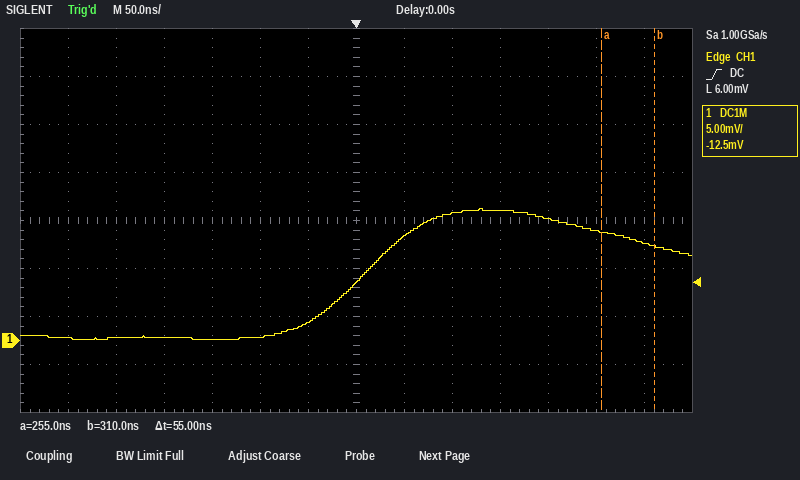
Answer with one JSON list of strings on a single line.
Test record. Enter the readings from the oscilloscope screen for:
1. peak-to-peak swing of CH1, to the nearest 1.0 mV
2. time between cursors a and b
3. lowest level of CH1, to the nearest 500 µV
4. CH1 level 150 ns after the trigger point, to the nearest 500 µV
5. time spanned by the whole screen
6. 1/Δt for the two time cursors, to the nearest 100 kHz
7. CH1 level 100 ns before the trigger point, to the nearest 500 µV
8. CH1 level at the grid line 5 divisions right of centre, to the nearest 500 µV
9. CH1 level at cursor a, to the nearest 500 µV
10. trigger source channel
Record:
["14.0 mV", "55 ns", "0.0 mV", "13.5 mV", "700 ns", "18.2 MHz", "500 µV", "11.5 mV", "11.5 mV", "CH1"]
